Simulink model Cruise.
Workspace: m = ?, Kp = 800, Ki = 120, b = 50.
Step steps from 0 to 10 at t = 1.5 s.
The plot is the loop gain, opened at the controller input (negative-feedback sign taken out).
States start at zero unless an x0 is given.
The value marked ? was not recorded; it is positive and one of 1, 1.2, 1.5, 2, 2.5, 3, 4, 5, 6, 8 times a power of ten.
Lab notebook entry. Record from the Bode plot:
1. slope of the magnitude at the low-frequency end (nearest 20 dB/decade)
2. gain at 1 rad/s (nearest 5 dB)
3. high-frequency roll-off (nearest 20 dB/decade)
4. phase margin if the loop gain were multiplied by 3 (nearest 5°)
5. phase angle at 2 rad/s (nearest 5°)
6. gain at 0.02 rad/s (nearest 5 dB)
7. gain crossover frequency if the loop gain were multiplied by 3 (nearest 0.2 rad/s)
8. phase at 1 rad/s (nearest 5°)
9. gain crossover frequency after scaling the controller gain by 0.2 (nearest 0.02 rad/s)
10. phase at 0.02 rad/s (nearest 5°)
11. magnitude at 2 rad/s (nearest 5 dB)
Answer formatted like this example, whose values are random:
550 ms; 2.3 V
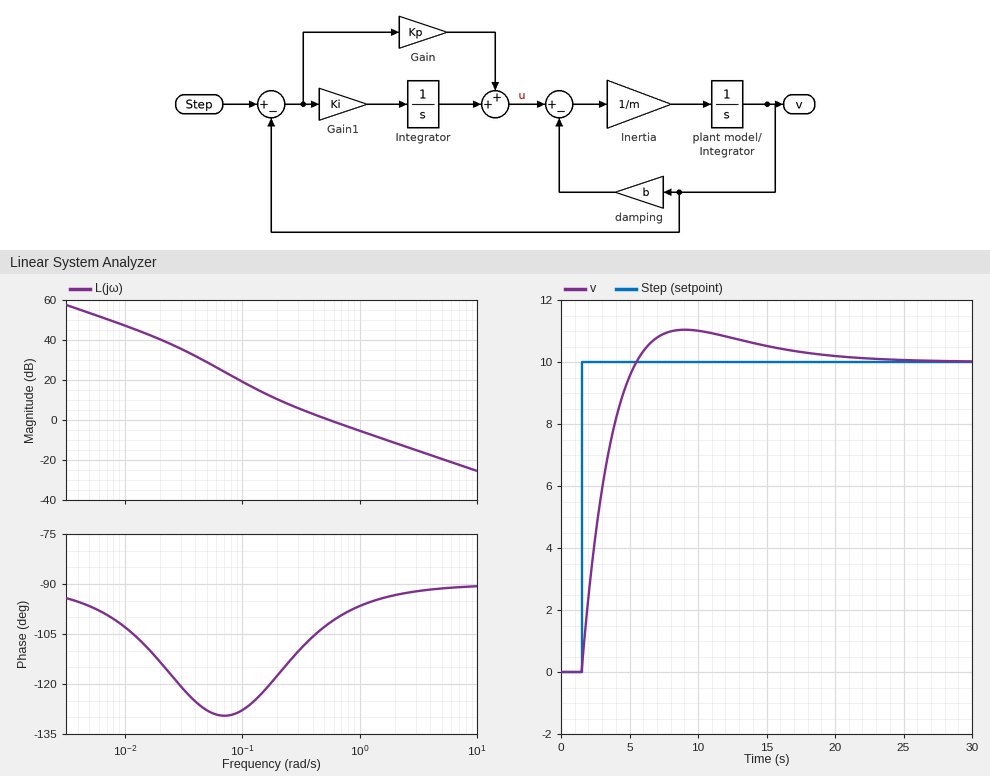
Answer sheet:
-20 dB/decade; -5 dB; -20 dB/decade; 85°; -95°; 40 dB; 1.6 rad/s; -95°; 0.14 rad/s; -115°; -10 dB
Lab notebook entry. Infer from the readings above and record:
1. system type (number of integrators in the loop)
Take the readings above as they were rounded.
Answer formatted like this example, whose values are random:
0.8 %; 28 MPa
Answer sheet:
1
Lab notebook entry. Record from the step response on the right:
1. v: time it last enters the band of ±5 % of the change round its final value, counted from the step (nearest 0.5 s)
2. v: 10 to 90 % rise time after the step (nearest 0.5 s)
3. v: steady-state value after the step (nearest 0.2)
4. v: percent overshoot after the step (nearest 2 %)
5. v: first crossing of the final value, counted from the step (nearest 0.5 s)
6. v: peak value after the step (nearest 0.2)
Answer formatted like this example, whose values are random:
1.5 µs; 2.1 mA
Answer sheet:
13.5 s; 3.0 s; 10.0; 10 %; 4.0 s; 11.0
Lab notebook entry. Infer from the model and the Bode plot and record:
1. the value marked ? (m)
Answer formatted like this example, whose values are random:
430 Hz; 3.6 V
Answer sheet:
1500
